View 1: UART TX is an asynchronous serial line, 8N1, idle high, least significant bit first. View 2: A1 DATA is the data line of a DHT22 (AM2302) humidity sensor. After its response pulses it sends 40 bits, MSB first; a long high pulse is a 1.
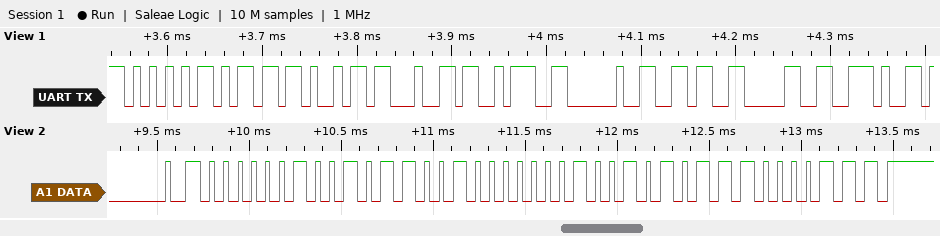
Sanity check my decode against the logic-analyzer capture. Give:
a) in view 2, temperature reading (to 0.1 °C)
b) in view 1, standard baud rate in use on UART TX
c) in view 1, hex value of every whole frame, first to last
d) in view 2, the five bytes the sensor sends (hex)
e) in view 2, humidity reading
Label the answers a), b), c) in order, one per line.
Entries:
a) 29.9 °C
b) 115200 baud
c) 55 6D 69 64 3A 20 36 30 2E
d) 02 59 01 2B 87
e) 60.1 %
